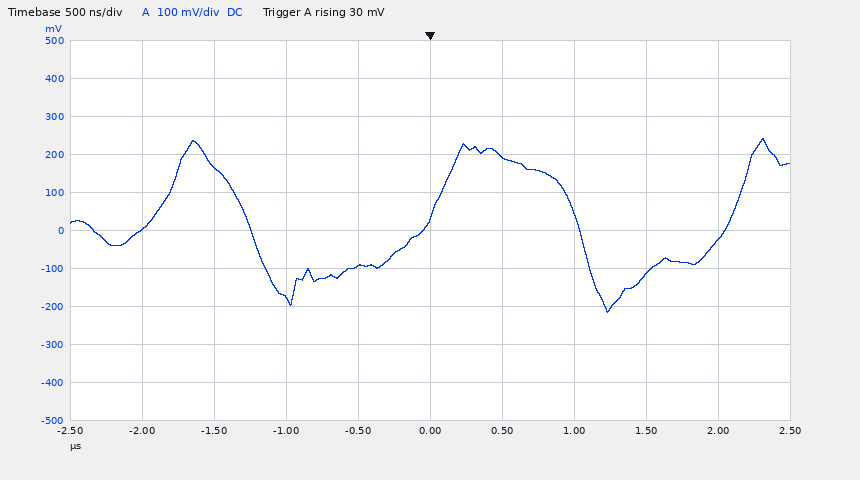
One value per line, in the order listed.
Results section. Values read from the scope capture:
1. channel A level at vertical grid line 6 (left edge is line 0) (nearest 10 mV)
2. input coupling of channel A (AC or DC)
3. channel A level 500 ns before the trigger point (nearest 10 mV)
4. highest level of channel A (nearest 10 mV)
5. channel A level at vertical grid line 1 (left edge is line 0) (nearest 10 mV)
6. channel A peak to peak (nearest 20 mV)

190 mV
DC
-90 mV
240 mV
0 mV
460 mV
